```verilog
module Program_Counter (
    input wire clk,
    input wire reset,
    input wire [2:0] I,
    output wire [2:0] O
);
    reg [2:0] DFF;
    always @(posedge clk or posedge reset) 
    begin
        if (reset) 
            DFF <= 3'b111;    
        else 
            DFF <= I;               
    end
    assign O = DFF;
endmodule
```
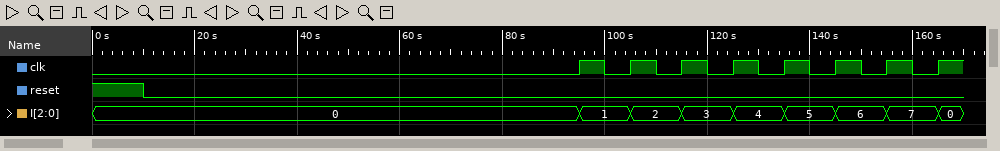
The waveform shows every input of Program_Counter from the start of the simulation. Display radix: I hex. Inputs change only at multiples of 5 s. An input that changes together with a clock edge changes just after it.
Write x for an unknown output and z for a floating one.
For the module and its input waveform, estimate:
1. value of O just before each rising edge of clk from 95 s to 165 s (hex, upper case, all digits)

7, 0, 1, 2, 3, 4, 5, 6
